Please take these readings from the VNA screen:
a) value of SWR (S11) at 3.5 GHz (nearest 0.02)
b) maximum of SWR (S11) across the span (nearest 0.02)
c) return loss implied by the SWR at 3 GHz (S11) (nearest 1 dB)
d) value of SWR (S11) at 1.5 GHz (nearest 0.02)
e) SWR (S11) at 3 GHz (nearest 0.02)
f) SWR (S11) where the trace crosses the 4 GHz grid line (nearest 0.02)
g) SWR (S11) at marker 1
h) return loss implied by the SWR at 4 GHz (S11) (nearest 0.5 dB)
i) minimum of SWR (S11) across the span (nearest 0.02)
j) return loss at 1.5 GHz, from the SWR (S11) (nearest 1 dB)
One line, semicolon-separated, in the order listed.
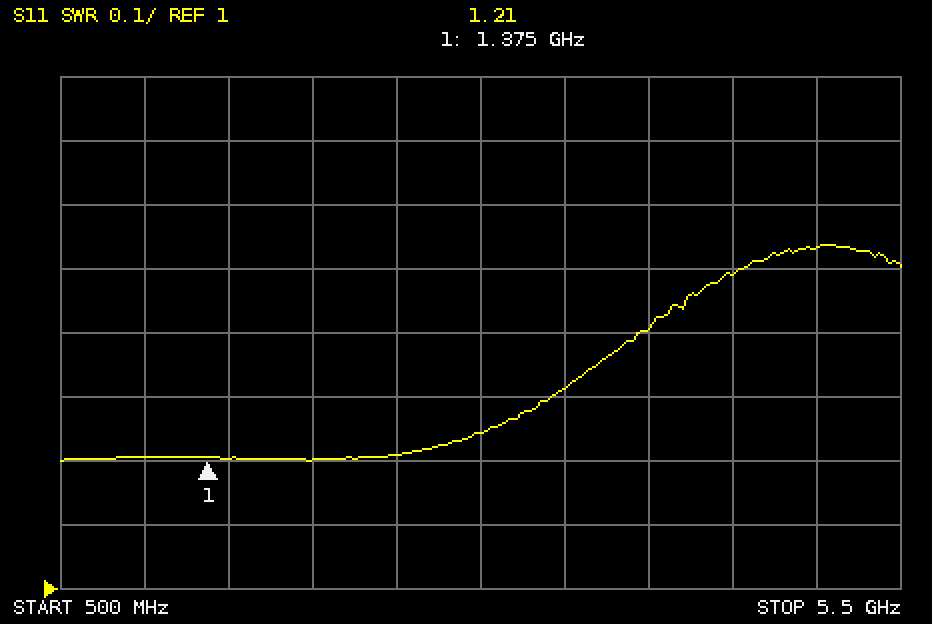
1.32; 1.54; 19 dB; 1.20; 1.24; 1.40; 1.21; 15.5 dB; 1.20; 21 dB
